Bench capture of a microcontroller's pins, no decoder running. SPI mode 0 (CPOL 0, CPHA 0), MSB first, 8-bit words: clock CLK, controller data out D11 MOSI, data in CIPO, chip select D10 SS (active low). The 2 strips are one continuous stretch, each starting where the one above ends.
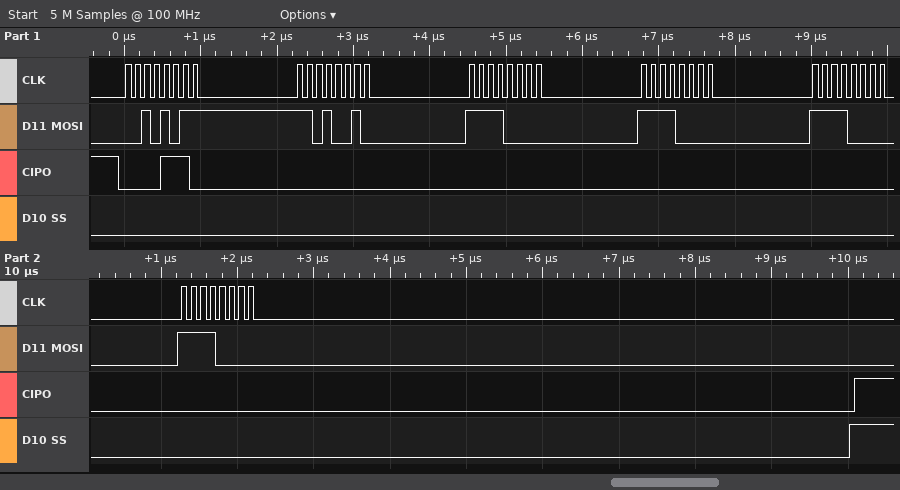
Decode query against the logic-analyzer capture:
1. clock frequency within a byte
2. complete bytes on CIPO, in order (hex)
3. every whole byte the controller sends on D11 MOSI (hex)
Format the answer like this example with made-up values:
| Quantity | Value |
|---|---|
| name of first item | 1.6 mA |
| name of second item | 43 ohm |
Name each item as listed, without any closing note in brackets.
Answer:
| Quantity | Value |
|---|---|
| clock frequency within a byte | 8 MHz |
| complete bytes on CIPO, in order | 0x0E 0x00 0x00 0x00 0x00 0x00 |
| every whole byte the controller sends on D11 MOSI | 0x2B 0xD2 0xF0 0xF0 0xF0 0xF0 |
